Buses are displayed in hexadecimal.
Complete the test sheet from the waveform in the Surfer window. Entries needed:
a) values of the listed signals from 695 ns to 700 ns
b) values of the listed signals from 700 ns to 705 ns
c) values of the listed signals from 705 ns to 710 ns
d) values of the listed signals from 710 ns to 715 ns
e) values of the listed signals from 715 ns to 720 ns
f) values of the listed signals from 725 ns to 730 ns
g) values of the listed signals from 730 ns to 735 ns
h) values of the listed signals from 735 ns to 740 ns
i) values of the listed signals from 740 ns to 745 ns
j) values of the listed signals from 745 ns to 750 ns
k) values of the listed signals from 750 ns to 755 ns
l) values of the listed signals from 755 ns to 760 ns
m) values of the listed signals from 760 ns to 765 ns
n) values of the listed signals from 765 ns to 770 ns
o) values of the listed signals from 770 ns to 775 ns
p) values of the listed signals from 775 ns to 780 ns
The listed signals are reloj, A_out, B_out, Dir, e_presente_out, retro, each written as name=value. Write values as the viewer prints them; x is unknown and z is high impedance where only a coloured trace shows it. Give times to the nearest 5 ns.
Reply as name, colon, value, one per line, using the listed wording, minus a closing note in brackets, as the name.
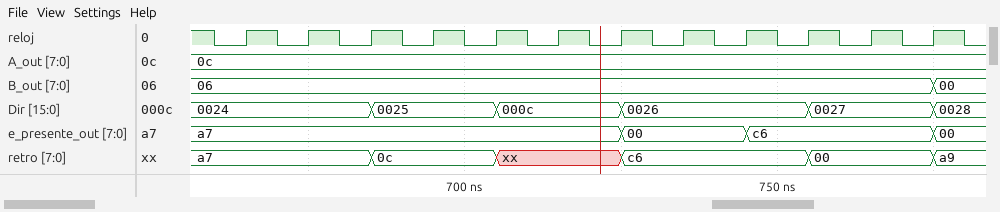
values of the listed signals from 695 ns to 700 ns: reloj=1, A_out=0c, B_out=06, Dir=0025, e_presente_out=a7, retro=0c
values of the listed signals from 700 ns to 705 ns: reloj=0, A_out=0c, B_out=06, Dir=0025, e_presente_out=a7, retro=0c
values of the listed signals from 705 ns to 710 ns: reloj=1, A_out=0c, B_out=06, Dir=000c, e_presente_out=a7, retro=xx
values of the listed signals from 710 ns to 715 ns: reloj=0, A_out=0c, B_out=06, Dir=000c, e_presente_out=a7, retro=xx
values of the listed signals from 715 ns to 720 ns: reloj=1, A_out=0c, B_out=06, Dir=000c, e_presente_out=a7, retro=xx
values of the listed signals from 725 ns to 730 ns: reloj=1, A_out=0c, B_out=06, Dir=0026, e_presente_out=00, retro=c6
values of the listed signals from 730 ns to 735 ns: reloj=0, A_out=0c, B_out=06, Dir=0026, e_presente_out=00, retro=c6
values of the listed signals from 735 ns to 740 ns: reloj=1, A_out=0c, B_out=06, Dir=0026, e_presente_out=00, retro=c6
values of the listed signals from 740 ns to 745 ns: reloj=0, A_out=0c, B_out=06, Dir=0026, e_presente_out=00, retro=c6
values of the listed signals from 745 ns to 750 ns: reloj=1, A_out=0c, B_out=06, Dir=0026, e_presente_out=c6, retro=c6
values of the listed signals from 750 ns to 755 ns: reloj=0, A_out=0c, B_out=06, Dir=0026, e_presente_out=c6, retro=c6
values of the listed signals from 755 ns to 760 ns: reloj=1, A_out=0c, B_out=06, Dir=0027, e_presente_out=c6, retro=00
values of the listed signals from 760 ns to 765 ns: reloj=0, A_out=0c, B_out=06, Dir=0027, e_presente_out=c6, retro=00
values of the listed signals from 765 ns to 770 ns: reloj=1, A_out=0c, B_out=06, Dir=0027, e_presente_out=c6, retro=00
values of the listed signals from 770 ns to 775 ns: reloj=0, A_out=0c, B_out=06, Dir=0027, e_presente_out=c6, retro=00
values of the listed signals from 775 ns to 780 ns: reloj=1, A_out=0c, B_out=00, Dir=0028, e_presente_out=00, retro=a9
